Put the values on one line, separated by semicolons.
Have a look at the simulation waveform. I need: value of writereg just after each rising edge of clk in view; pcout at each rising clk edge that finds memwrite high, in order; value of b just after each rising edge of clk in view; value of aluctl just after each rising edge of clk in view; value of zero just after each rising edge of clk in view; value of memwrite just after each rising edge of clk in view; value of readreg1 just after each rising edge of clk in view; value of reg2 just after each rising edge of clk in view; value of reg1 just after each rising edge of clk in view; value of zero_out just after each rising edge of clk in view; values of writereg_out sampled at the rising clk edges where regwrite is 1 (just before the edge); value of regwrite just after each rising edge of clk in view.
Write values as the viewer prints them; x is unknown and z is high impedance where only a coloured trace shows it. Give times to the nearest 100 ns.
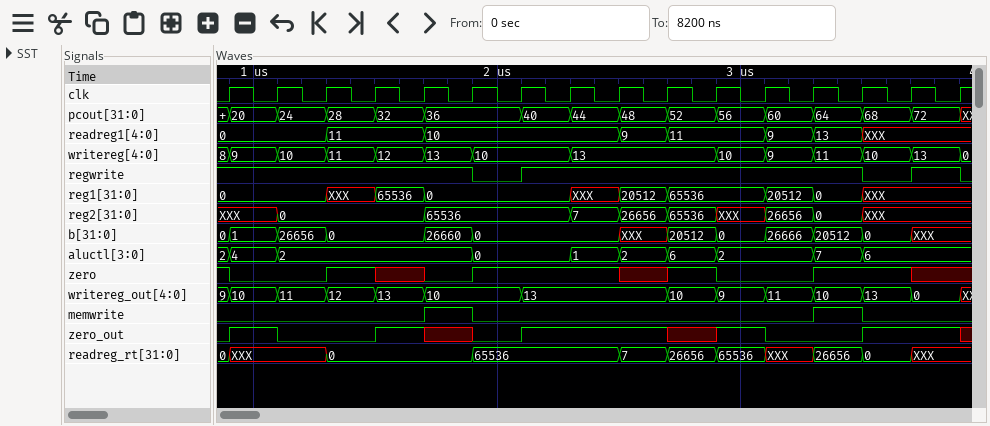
9, 10, 11, 12, 13, 10, 10, 13, 13, 13, 10, 9, 11, 10, 13, 0; 36, 64; 1, 26656, 0, 0, 26660, 0, 0, 0, XXX, 20512, 0, 26666, 20512, 0, XXX, XXX; 4, 2, 2, 2, 2, 0, 0, 1, 2, 6, 2, 2, 7, 6, 6, 6; 0 0 1 x 0 1 1 1 x 1 0 0 1 1 x x; 0 0 0 0 1 0 0 0 0 0 0 0 1 0 0 0; 0, 0, 11, 11, 10, 10, 10, 10, 9, 11, 11, 9, 13, XXX, XXX, XXX; XXX, 0, 0, 0, 65536, 65536, 65536, 7, 26656, 65536, XXX, 26656, 0, XXX, XXX, XXX; 0, 0, XXX, 65536, 0, 0, 0, XXX, 20512, 65536, 65536, 20512, 0, XXX, XXX, XXX; 1 0 0 1 x 0 1 1 1 x 1 0 0 1 1 x; 9, 10, 11, 12, 13, 10, 13, 13, 13, 10, 9, 11, 10, 0; 1 1 1 1 1 0 1 1 1 1 1 1 1 0 1 0
